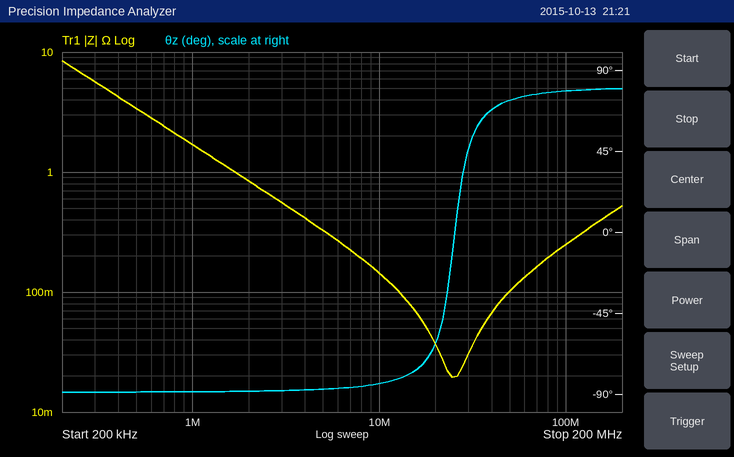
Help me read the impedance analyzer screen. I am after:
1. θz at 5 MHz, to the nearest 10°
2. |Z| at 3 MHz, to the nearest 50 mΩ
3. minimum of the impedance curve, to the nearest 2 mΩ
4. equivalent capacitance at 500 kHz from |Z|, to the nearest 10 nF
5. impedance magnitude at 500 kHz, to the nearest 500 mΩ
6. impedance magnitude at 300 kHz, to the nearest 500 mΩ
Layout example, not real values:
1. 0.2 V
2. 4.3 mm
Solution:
1. -90°
2. 550 mΩ
3. 20 mΩ
4. 90 nF
5. 3.5 Ω
6. 5.5 Ω
